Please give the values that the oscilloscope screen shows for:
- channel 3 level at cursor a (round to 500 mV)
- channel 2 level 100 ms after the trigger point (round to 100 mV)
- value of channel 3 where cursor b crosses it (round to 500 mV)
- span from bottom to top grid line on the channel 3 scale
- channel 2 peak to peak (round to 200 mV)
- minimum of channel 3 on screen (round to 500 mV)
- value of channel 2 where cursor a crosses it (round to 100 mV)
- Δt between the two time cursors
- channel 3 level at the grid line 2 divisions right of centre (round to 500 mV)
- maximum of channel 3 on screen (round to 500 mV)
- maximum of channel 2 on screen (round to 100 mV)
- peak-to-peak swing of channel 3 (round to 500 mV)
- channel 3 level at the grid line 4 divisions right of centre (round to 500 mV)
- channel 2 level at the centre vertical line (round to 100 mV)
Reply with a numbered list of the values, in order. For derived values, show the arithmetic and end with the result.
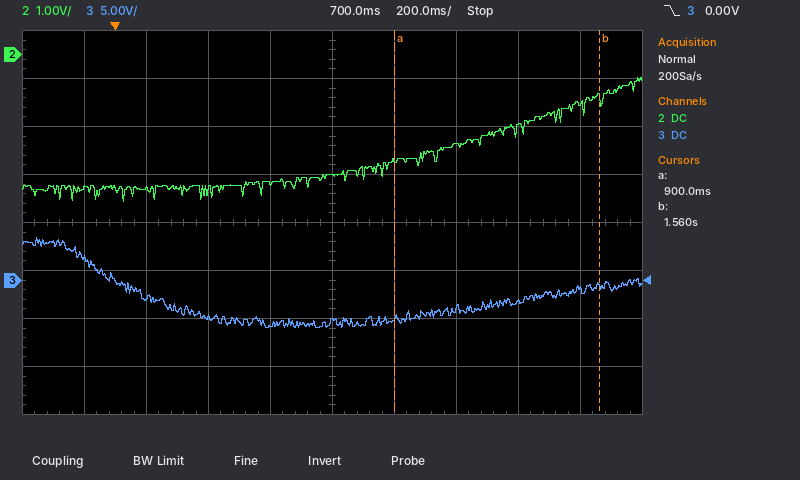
1. -4.0 V
2. -2.8 V
3. -500 mV
4. 40 V
5. 2.6 V
6. -5.0 V
7. -2.2 V
8. 1.56 s − (900 ms) = 660 ms
9. -3.0 V
10. 4.5 V
11. -500 mV
12. 4.5 V − (-5.0 V) = 9.5 V
13. -1.0 V
14. -2.5 V
